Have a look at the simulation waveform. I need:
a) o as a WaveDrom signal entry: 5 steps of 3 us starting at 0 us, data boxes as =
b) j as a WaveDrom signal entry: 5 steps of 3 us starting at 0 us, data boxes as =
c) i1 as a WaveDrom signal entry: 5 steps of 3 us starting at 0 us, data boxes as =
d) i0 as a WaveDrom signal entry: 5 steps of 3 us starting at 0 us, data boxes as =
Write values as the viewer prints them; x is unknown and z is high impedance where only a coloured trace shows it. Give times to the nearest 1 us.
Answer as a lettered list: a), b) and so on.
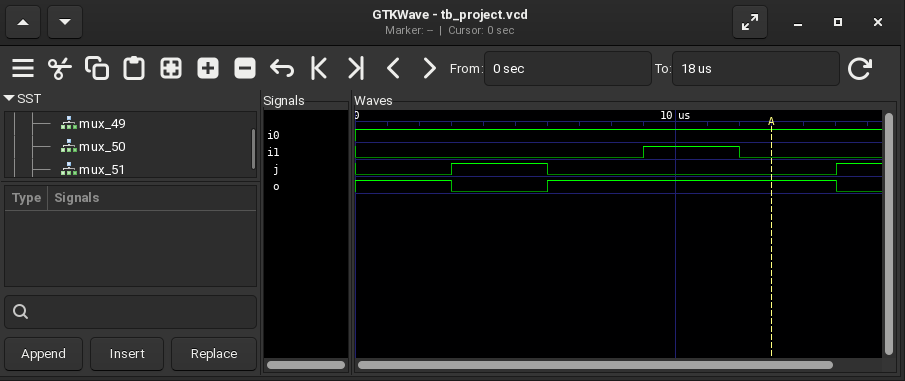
a) {name: 'o', wave: '101..'}
b) {name: 'j', wave: '010..'}
c) {name: 'i1', wave: '0..10'}
d) {name: 'i0', wave: '1....'}
